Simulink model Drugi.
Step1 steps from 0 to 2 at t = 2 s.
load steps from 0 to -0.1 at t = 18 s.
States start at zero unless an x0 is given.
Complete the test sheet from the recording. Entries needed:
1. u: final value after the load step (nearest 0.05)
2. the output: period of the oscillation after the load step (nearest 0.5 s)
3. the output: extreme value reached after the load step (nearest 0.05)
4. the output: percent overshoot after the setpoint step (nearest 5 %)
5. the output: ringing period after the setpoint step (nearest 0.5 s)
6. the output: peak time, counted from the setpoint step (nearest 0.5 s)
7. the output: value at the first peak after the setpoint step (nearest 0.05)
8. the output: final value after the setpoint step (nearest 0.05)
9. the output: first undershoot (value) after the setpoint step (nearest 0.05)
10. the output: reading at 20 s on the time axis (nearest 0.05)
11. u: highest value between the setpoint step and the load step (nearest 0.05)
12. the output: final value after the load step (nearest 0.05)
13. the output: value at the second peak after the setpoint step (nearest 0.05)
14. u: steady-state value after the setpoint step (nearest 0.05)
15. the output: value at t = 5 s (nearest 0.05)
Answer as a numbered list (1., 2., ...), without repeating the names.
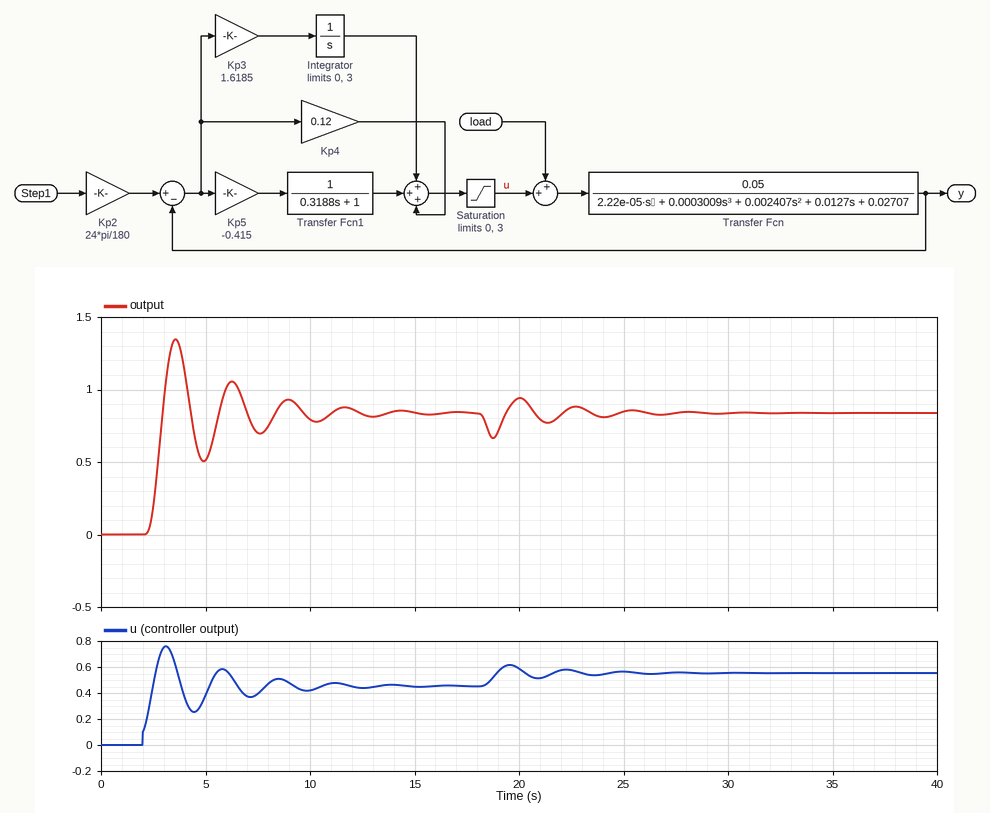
1. 0.55
2. 2.5 s
3. 0.65
4. 60 %
5. 2.5 s
6. 1.5 s
7. 1.35
8. 0.85
9. 0.50
10. 0.95
11. 0.75
12. 0.85
13. 1.05
14. 0.45
15. 0.50
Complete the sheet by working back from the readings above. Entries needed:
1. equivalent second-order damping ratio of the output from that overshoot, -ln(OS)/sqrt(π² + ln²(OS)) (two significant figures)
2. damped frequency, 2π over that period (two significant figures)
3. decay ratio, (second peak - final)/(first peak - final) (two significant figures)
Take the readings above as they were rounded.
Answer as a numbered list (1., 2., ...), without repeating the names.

1. 0.16
2. 2.5 rad/s
3. 0.40
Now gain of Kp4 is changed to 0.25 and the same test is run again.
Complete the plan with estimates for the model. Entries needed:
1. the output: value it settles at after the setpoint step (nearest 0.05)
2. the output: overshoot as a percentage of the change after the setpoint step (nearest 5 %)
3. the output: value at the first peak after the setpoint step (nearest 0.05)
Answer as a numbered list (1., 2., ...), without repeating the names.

1. 0.85
2. 35 %
3. 1.15
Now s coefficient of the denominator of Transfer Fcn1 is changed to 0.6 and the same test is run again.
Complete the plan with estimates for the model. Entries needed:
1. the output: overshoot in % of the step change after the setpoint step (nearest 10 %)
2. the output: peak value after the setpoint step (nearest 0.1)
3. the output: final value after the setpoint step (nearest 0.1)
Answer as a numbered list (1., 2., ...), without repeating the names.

1. 40 %
2. 1.2
3. 0.8
